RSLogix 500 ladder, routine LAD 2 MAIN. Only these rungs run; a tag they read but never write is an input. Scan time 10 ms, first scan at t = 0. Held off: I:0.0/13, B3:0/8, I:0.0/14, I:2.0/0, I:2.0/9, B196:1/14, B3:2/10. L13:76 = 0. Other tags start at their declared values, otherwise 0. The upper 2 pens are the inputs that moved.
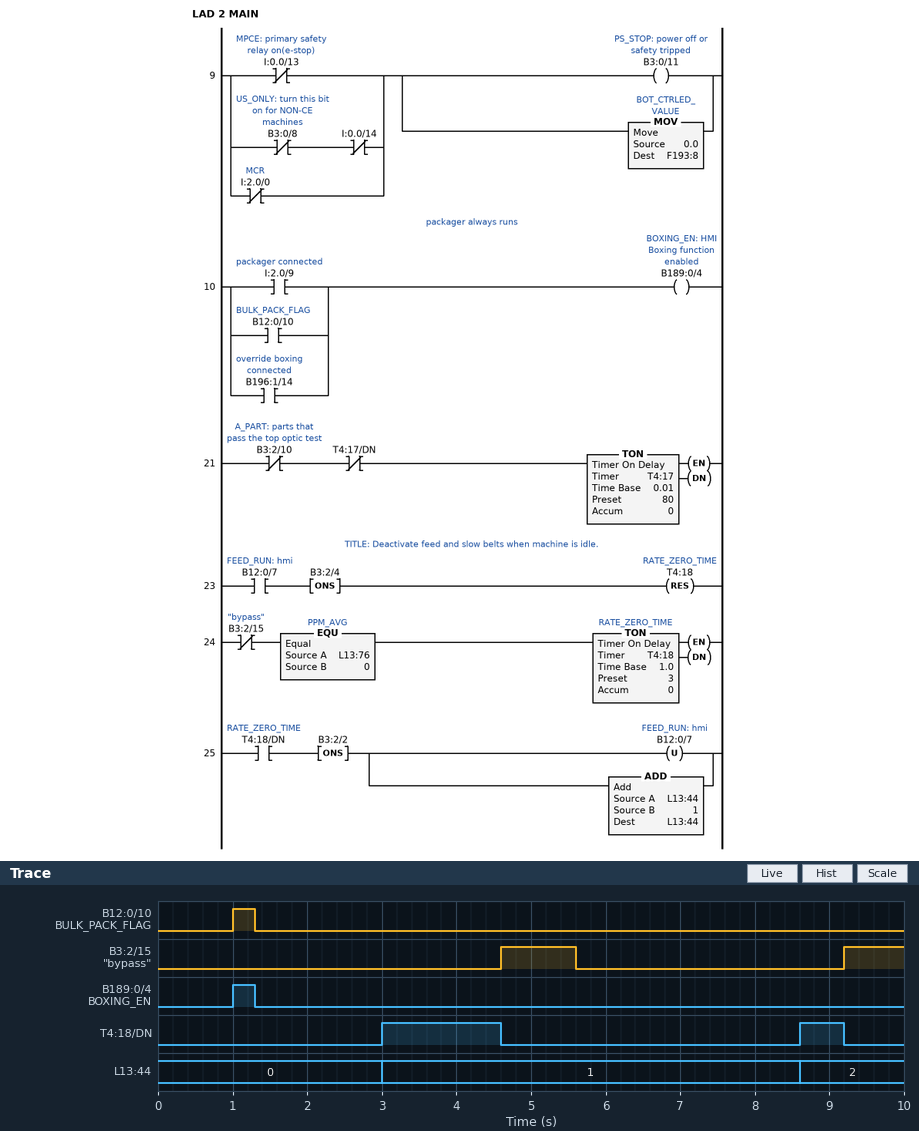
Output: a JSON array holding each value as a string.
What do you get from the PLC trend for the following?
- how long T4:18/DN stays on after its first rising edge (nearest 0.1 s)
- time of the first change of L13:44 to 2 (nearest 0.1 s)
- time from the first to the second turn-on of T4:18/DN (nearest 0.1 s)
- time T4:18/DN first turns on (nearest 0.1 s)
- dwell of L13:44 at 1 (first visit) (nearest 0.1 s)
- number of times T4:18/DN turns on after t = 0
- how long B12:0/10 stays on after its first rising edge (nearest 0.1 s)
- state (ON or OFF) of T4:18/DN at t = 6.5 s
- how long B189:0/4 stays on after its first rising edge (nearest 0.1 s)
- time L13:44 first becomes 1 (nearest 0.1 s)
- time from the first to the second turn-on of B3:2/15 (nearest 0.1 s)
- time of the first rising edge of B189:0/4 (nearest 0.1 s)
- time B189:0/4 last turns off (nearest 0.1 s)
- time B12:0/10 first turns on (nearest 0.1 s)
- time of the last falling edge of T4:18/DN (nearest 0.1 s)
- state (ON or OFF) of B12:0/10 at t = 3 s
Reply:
["1.6 s", "8.6 s", "5.6 s", "3.0 s", "5.6 s", "2", "0.3 s", "OFF", "0.3 s", "3.0 s", "4.6 s", "1.0 s", "1.3 s", "1.0 s", "9.2 s", "OFF"]
